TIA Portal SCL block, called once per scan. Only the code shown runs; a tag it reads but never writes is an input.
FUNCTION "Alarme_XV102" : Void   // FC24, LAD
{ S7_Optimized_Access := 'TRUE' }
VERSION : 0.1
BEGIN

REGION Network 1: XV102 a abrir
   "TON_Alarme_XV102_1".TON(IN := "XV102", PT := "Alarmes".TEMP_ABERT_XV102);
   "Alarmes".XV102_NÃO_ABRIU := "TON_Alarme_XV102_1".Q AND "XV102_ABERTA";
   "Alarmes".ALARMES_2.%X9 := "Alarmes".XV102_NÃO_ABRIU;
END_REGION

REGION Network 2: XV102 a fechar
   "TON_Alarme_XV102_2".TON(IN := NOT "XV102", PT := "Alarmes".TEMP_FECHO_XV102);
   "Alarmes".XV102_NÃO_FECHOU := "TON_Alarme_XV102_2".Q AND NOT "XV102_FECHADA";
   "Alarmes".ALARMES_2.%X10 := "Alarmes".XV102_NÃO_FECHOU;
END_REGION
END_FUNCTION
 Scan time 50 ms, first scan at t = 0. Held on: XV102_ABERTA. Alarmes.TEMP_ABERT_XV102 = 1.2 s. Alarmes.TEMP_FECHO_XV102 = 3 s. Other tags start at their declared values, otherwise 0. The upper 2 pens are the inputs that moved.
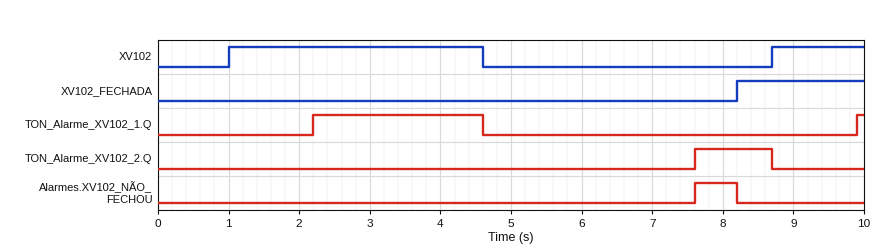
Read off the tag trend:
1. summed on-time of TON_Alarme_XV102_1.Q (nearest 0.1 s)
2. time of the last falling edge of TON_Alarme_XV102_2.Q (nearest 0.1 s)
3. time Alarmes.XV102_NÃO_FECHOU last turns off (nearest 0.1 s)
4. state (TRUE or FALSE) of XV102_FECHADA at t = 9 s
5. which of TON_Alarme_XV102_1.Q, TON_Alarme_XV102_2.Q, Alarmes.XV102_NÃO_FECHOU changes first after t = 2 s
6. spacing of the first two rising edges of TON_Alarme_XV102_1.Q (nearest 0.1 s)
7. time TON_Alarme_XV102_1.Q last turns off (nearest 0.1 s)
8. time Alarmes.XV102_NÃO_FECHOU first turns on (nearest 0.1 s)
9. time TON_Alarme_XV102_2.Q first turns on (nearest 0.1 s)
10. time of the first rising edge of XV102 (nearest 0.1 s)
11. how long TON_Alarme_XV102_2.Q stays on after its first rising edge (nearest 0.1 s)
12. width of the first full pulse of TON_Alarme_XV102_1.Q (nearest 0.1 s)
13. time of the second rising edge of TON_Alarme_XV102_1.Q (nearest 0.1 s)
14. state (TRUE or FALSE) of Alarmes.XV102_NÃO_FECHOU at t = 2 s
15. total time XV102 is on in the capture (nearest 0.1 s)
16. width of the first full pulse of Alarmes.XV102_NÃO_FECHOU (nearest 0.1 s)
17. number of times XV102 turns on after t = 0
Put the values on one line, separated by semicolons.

2.5 s; 8.7 s; 8.2 s; TRUE; TON_Alarme_XV102_1.Q; 7.7 s; 4.6 s; 7.6 s; 7.6 s; 1.0 s; 1.1 s; 2.4 s; 9.9 s; FALSE; 4.9 s; 0.6 s; 2
